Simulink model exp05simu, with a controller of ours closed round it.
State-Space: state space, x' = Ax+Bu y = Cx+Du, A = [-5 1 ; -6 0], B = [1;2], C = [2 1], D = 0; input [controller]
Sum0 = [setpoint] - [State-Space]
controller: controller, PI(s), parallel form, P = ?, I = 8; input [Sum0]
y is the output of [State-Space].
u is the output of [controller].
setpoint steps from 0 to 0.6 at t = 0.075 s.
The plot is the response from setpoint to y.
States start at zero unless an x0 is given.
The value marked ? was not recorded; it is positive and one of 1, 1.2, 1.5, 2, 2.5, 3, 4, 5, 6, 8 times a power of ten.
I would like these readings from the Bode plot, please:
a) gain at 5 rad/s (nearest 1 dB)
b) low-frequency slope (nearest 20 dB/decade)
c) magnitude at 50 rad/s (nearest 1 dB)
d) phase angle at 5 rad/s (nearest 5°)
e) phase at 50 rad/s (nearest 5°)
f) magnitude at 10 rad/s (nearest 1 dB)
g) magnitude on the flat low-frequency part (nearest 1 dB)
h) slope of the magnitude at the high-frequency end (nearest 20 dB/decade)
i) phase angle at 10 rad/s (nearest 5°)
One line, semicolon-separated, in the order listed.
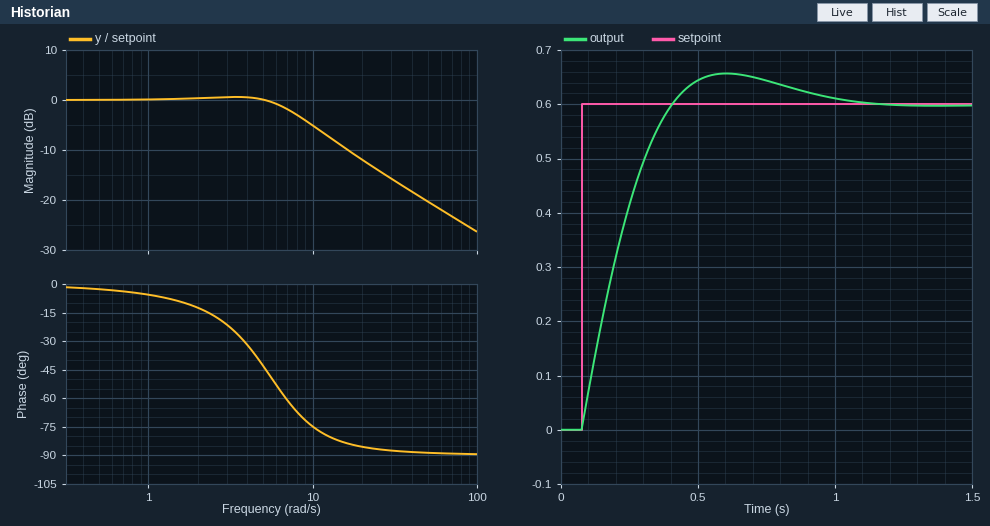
0 dB; 0 dB/decade; -20 dB; -45°; -90°; -5 dB; 0 dB; -20 dB/decade; -75°
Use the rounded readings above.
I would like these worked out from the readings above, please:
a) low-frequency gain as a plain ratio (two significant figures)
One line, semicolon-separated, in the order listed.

1.0
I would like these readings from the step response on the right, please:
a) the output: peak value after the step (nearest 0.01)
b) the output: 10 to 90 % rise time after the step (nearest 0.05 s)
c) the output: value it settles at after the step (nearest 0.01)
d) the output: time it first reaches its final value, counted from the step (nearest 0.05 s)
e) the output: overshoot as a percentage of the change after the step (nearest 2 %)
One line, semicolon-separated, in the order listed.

0.66; 0.25 s; 0.60; 0.35 s; 10 %
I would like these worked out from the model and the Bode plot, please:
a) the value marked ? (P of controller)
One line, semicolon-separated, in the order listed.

1.2
